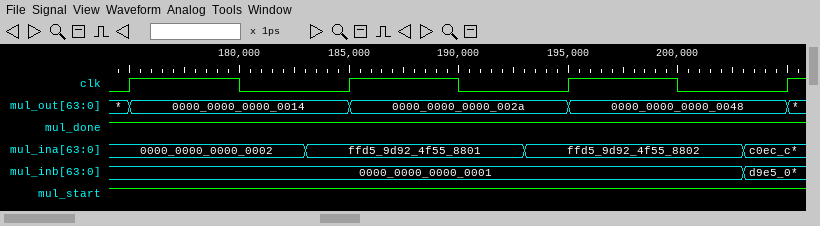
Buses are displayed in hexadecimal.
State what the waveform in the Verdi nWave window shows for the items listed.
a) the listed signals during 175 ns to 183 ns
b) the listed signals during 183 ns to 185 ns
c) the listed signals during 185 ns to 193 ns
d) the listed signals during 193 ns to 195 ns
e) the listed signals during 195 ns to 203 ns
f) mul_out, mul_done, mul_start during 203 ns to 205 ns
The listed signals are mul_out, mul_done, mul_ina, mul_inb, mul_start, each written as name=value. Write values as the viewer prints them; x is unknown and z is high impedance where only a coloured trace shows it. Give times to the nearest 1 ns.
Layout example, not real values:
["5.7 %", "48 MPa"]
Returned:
["mul_out=0000_0000_0000_0014, mul_done=1, mul_ina=0000_0000_0000_0002, mul_inb=0000_0000_0000_0001, mul_start=1", "mul_out=0000_0000_0000_0014, mul_done=1, mul_ina=ffd5_9d92_4f55_8801, mul_inb=0000_0000_0000_0001, mul_start=1", "mul_out=0000_0000_0000_002a, mul_done=1, mul_ina=ffd5_9d92_4f55_8801, mul_inb=0000_0000_0000_0001, mul_start=1", "mul_out=0000_0000_0000_002a, mul_done=1, mul_ina=ffd5_9d92_4f55_8802, mul_inb=0000_0000_0000_0001, mul_start=1", "mul_out=0000_0000_0000_0048, mul_done=1, mul_ina=ffd5_9d92_4f55_8802, mul_inb=0000_0000_0000_0001, mul_start=1", "mul_out=0000_0000_0000_0048, mul_done=1, mul_start=1"]
